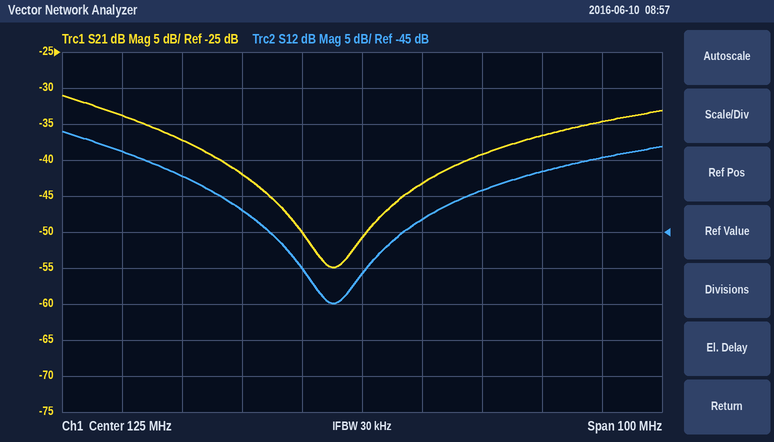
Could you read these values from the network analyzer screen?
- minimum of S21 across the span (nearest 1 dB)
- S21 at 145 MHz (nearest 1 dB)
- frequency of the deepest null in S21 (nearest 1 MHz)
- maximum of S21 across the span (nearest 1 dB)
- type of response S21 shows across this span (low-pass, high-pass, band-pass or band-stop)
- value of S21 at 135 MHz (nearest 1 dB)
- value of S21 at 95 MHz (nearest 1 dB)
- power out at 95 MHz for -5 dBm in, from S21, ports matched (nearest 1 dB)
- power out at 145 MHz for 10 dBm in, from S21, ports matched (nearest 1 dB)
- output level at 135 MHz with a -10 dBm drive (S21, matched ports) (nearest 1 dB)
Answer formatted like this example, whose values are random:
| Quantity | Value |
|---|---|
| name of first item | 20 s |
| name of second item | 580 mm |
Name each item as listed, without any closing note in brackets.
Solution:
| Quantity | Value |
|---|---|
| minimum of S21 across the span | -55 dB |
| S21 at 145 MHz | -39 dB |
| frequency of the deepest null in S21 | 120 MHz |
| maximum of S21 across the span | -31 dB |
| type of response S21 shows across this span | band-stop |
| value of S21 at 135 MHz | -43 dB |
| value of S21 at 95 MHz | -37 dB |
| power out at 95 MHz for -5 dBm in, from S21, ports matched | -42 dBm |
| power out at 145 MHz for 10 dBm in, from S21, ports matched | -29 dBm |
| output level at 135 MHz with a -10 dBm drive (S21, matched ports) | -53 dBm |
